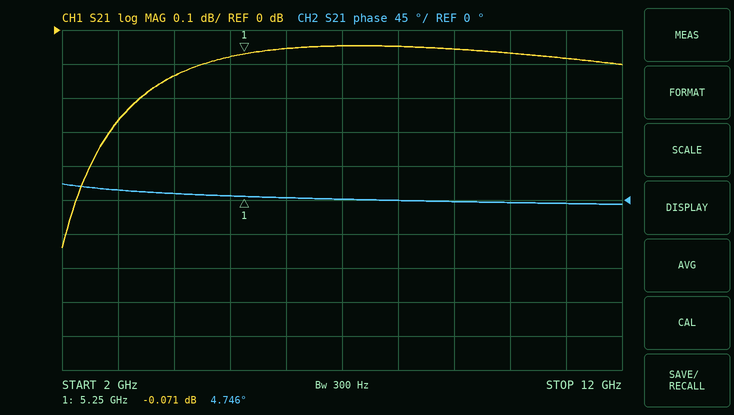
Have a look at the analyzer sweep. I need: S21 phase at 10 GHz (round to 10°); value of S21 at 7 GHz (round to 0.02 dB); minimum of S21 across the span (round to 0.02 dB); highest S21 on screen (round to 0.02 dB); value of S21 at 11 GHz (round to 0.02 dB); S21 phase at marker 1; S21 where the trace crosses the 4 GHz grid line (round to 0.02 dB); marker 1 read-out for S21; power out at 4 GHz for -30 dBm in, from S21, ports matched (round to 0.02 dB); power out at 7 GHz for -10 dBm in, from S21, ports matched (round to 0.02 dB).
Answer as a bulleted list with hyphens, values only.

- 0°
- -0.04 dB
- -0.64 dB
- -0.04 dB
- -0.08 dB
- 4.746°
- -0.14 dB
- -0.071 dB
- -30.14 dBm
- -10.04 dBm
